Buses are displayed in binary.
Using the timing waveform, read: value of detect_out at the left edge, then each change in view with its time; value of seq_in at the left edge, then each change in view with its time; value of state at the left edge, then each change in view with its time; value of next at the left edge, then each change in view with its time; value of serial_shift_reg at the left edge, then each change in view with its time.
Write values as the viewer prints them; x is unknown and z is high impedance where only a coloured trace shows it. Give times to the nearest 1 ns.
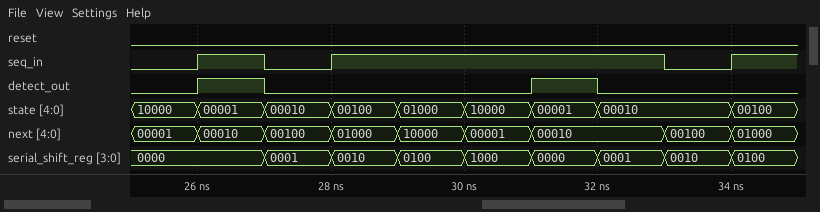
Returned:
0, 1 at 26 ns, 0 at 27 ns, 1 at 31 ns, 0 at 32 ns
0, 1 at 26 ns, 0 at 27 ns, 1 at 28 ns, 0 at 33 ns, 1 at 34 ns
10000, 00001 at 26 ns, 00010 at 27 ns, 00100 at 28 ns, 01000 at 29 ns, 10000 at 30 ns, 00001 at 31 ns, 00010 at 32 ns, 00100 at 34 ns
00001, 00010 at 26 ns, 00100 at 27 ns, 01000 at 28 ns, 10000 at 29 ns, 00001 at 30 ns, 00010 at 31 ns, 00100 at 33 ns, 01000 at 34 ns
0000, 0001 at 27 ns, 0010 at 28 ns, 0100 at 29 ns, 1000 at 30 ns, 0000 at 31 ns, 0001 at 32 ns, 0010 at 33 ns, 0100 at 34 ns
